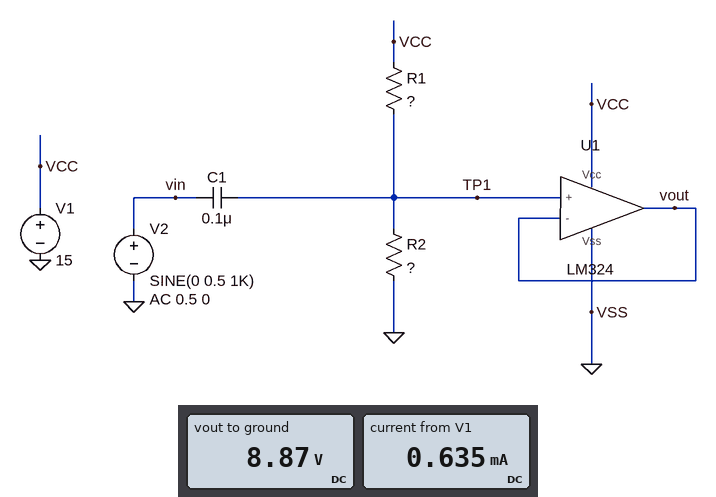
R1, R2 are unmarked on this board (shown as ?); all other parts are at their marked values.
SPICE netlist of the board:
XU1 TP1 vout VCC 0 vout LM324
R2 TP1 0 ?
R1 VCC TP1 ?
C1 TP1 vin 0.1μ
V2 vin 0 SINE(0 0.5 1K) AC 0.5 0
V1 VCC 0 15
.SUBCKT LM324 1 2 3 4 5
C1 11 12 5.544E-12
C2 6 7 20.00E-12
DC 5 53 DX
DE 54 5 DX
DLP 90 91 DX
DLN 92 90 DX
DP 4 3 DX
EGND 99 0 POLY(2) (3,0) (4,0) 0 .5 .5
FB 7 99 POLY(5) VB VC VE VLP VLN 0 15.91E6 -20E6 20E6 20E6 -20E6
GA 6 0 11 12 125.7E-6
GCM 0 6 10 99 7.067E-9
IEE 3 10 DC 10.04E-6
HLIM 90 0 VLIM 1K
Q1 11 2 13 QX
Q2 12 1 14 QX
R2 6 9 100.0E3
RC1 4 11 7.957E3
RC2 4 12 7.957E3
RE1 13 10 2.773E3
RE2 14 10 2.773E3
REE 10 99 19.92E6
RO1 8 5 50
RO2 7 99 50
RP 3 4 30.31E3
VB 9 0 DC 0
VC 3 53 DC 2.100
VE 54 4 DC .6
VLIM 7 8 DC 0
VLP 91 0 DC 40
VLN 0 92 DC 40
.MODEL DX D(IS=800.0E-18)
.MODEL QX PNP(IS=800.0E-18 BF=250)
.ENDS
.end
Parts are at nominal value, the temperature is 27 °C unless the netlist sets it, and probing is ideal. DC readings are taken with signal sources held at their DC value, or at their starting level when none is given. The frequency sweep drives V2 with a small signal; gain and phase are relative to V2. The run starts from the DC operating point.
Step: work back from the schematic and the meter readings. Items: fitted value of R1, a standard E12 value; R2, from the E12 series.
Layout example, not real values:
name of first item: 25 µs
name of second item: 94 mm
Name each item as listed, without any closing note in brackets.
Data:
fitted value of R1, a standard E12 value: 47 kΩ
R2, from the E12 series: 68 kΩ
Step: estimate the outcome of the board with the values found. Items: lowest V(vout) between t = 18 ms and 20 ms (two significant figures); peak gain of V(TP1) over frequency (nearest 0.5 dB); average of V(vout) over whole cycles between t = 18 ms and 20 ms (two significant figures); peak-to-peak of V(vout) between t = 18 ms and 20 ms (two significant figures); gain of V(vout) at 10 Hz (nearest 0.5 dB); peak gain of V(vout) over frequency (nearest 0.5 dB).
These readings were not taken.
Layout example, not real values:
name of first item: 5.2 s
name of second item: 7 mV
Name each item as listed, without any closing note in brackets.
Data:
lowest V(vout) between t = 18 ms and 20 ms: 8.4 V
peak gain of V(TP1) over frequency: 0 dB
average of V(vout) over whole cycles between t = 18 ms and 20 ms: 8.9 V
peak-to-peak of V(vout) between t = 18 ms and 20 ms: 1.0 V
gain of V(vout) at 10 Hz: -15.5 dB
peak gain of V(vout) over frequency: 0 dB
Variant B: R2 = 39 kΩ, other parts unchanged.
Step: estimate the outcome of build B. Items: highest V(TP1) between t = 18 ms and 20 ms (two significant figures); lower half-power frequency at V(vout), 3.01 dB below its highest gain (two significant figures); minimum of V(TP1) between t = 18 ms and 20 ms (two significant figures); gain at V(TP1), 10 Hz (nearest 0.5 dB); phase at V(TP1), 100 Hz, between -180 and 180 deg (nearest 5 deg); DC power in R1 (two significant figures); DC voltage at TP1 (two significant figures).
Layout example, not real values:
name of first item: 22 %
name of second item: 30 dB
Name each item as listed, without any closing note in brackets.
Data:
highest V(TP1) between t = 18 ms and 20 ms: 7.3 V
lower half-power frequency at V(vout), 3.01 dB below its highest gain: 75 Hz
minimum of V(TP1) between t = 18 ms and 20 ms: 6.3 V
gain at V(TP1), 10 Hz: -17.5 dB
phase at V(TP1), 100 Hz, between -180 and 180 deg: 35 deg
DC power in R1: 1.4 mW
DC voltage at TP1: 6.8 V
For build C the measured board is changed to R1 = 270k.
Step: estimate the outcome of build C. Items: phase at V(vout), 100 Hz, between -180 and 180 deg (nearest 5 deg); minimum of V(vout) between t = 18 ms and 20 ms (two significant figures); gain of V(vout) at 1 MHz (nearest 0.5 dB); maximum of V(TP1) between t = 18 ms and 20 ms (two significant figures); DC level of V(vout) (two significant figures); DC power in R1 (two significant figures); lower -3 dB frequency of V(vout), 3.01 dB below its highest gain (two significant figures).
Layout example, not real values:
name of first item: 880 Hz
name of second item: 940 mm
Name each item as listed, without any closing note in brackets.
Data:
phase at V(vout), 100 Hz, between -180 and 180 deg: 15 deg
minimum of V(vout) between t = 18 ms and 20 ms: 2.5 V
gain of V(vout) at 1 MHz: -0.5 dB
maximum of V(TP1) between t = 18 ms and 20 ms: 3.5 V
DC level of V(vout): 3.0 V
DC power in R1: 530 µW
lower -3 dB frequency of V(vout), 3.01 dB below its highest gain: 30 Hz
